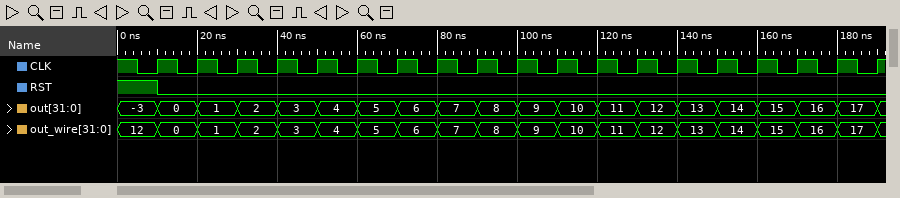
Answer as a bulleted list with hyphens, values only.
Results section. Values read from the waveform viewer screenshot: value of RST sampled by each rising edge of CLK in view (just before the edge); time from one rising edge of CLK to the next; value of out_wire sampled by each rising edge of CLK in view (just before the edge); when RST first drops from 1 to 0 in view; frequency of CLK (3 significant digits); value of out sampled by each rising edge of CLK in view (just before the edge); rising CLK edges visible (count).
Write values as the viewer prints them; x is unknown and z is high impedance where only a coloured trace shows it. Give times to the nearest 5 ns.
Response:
- 1 0 0 0 0 0 0 0 0 0 0 0 0 0 0 0 0 0 0
- 10 ns
- 12, 0, 1, 2, 3, 4, 5, 6, 7, 8, 9, 10, 11, 12, 13, 14, 15, 16, 17
- 10 ns
- 100 MHz
- -3, 0, 1, 2, 3, 4, 5, 6, 7, 8, 9, 10, 11, 12, 13, 14, 15, 16, 17
- 19
